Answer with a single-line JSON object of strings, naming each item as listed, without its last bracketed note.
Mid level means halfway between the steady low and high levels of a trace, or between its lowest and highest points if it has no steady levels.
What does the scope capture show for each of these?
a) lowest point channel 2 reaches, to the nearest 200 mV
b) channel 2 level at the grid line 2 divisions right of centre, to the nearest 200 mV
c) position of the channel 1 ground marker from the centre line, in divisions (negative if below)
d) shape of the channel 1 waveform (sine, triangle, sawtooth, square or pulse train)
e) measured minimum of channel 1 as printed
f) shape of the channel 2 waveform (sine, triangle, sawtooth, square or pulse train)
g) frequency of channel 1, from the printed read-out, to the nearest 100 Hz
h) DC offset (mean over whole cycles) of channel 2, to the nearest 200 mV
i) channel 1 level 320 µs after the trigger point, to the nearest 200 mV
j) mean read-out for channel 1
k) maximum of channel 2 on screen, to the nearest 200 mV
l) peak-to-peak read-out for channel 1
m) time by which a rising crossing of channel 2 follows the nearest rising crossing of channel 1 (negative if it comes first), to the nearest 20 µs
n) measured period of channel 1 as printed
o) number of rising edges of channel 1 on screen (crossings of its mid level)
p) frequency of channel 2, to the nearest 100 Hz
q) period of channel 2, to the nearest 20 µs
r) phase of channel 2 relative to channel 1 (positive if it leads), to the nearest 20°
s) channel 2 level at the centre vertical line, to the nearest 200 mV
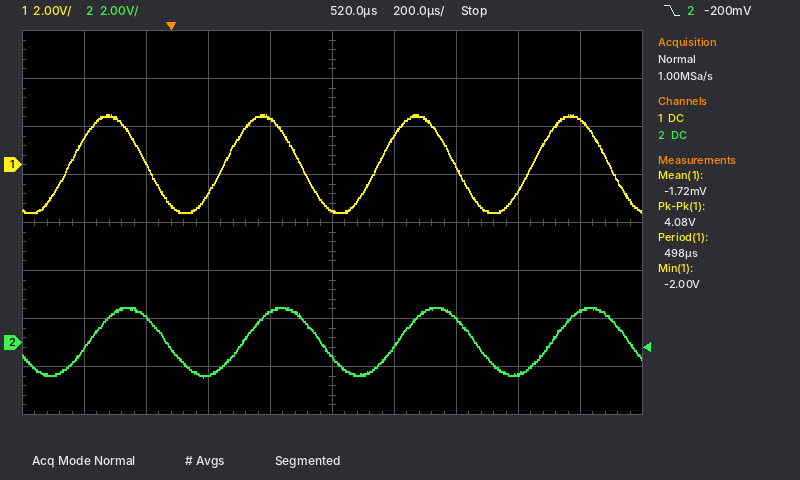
{"lowest point channel 2 reaches, to the nearest 200 mV": "-1.4 V", "channel 2 level at the grid line 2 divisions right of centre, to the nearest 200 mV": "1.0 V", "position of the channel 1 ground marker from the centre line, in divisions": "+1.2 div", "shape of the channel 1 waveform": "sine", "measured minimum of channel 1 as printed": "-2.00 V", "shape of the channel 2 waveform": "sine", "frequency of channel 1, from the printed read-out, to the nearest 100 Hz": "2.0 kHz", "DC offset (mean over whole cycles) of channel 2, to the nearest 200 mV": "0.0 V", "channel 1 level 320 µs after the trigger point, to the nearest 200 mV": "2.0 V", "mean read-out for channel 1": "-1.72 mV", "maximum of channel 2 on screen, to the nearest 200 mV": "1.4 V", "peak-to-peak read-out for channel 1": "4.08 V", "time by which a rising crossing of channel 2 follows the nearest rising crossing of channel 1 (negative if it comes first), to the nearest 20 µs": "+60 µs", "measured period of channel 1 as printed": "498 µs", "number of rising edges of channel 1 on screen": "4", "frequency of channel 2, to the nearest 100 Hz": "2.0 kHz", "period of channel 2, to the nearest 20 µs": "500 µs", "phase of channel 2 relative to channel 1 (positive if it leads), to the nearest 20°": "-40°", "channel 2 level at the centre vertical line, to the nearest 200 mV": "-600 mV"}
